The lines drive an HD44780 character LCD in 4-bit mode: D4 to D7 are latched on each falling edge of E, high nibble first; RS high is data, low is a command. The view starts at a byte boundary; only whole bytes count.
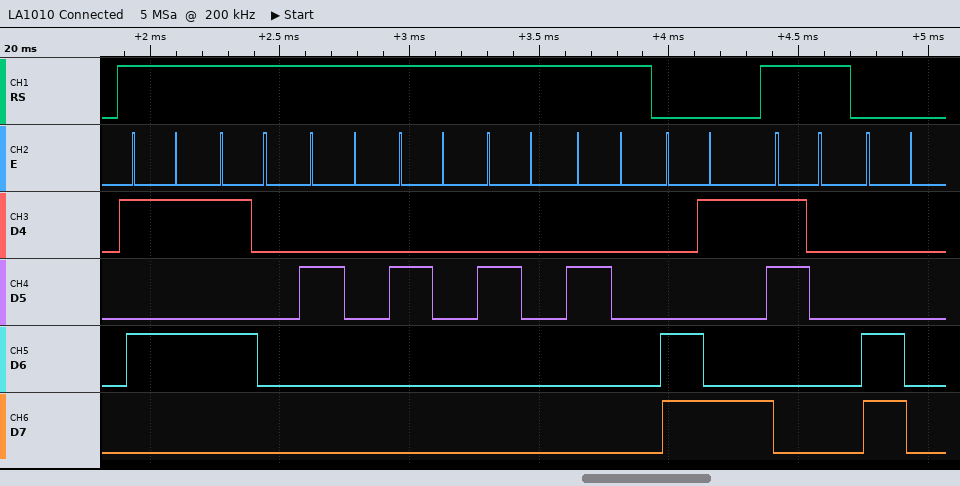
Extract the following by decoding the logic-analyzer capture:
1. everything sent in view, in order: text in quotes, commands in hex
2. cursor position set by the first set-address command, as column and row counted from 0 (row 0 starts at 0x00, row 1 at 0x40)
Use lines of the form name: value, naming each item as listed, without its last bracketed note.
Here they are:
everything sent in view, in order: text in quotes, commands in hex: "UP    " 0xC9 "0" 0xC0
cursor position set by the first set-address command, as column and row counted from 0: column 9, row 1
